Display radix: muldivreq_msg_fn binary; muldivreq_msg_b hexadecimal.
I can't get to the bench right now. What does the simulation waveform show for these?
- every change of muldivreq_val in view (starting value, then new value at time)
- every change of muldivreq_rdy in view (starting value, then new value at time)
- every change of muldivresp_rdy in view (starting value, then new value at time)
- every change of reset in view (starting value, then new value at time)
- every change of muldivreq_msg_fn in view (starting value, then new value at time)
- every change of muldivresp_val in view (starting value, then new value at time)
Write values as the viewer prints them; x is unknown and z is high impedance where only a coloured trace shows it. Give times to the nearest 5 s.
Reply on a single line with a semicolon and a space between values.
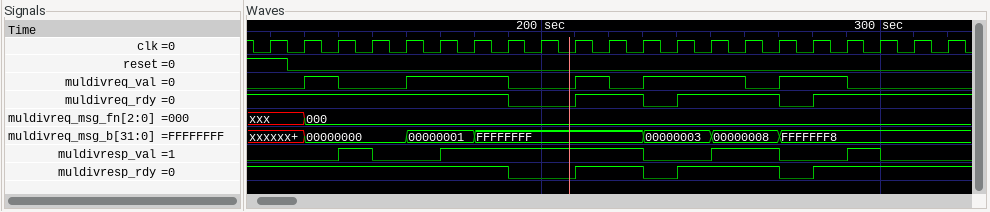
0, 1 at 130 s, 0 at 140 s, 1 at 160 s, 0 at 190 s, 1 at 210 s, 0 at 220 s, 1 at 230 s, 0 at 260 s, 1 at 270 s, 0 at 290 s; 1, 0 at 190 s, 1 at 210 s, 0 at 230 s, 1 at 240 s, 0 at 270 s, 1 at 280 s; 1, 0 at 190 s, 1 at 210 s, 0 at 230 s, 1 at 240 s, 0 at 270 s, 1 at 280 s; 1, 0 at 125 s; xxx, 000 at 130 s; 0, 1 at 140 s, 0 at 150 s, 1 at 170 s, 0 at 230 s, 1 at 250 s, 0 at 270 s, 1 at 290 s, 0 at 300 s
